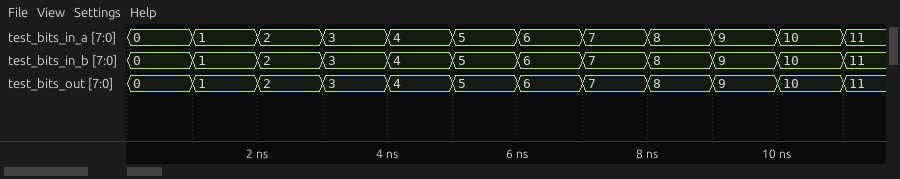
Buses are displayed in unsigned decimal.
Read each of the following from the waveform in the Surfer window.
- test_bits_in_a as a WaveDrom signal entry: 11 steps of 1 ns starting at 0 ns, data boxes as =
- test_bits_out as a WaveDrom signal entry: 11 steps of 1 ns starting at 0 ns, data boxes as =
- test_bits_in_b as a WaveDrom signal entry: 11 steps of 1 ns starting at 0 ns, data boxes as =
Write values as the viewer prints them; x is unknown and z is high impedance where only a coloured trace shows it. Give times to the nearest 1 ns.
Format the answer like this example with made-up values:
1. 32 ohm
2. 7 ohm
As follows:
1. {name: 'test_bits_in_a', wave: '===========', data: '0 1 2 3 4 5 6 7 8 9 10'}
2. {name: 'test_bits_out', wave: '===========', data: '0 1 2 3 4 5 6 7 8 9 10'}
3. {name: 'test_bits_in_b', wave: '===========', data: '0 1 2 3 4 5 6 7 8 9 10'}
